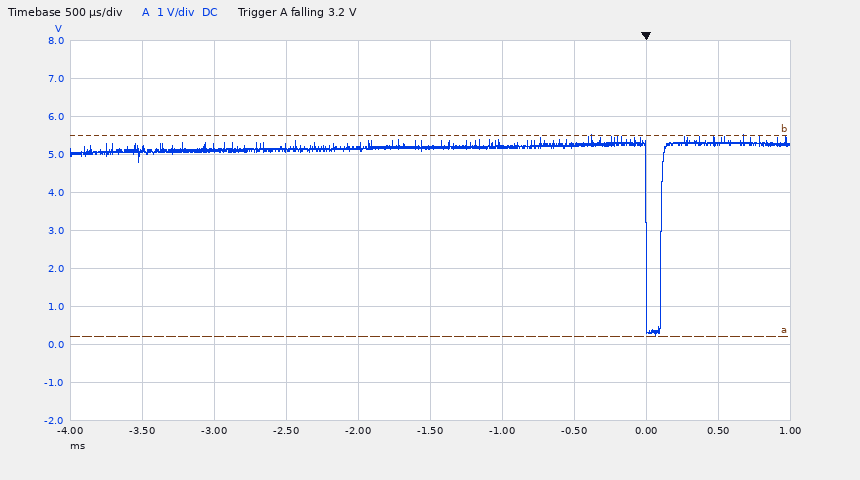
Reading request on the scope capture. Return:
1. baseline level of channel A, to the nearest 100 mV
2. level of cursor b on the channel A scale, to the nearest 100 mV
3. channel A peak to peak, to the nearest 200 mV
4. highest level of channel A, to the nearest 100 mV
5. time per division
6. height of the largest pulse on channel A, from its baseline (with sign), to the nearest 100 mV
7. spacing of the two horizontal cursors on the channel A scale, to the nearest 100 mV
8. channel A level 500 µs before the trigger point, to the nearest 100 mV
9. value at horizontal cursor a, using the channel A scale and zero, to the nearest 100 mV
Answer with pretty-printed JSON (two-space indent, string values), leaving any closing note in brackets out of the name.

{
  "baseline level of channel A, to the nearest 100 mV": "5.2 V",
  "level of cursor b on the channel A scale, to the nearest 100 mV": "5.5 V",
  "channel A peak to peak, to the nearest 200 mV": "5.2 V",
  "highest level of channel A, to the nearest 100 mV": "5.5 V",
  "time per division": "500 µs",
  "height of the largest pulse on channel A, from its baseline (with sign), to the nearest 100 mV": "-4.9 V",
  "spacing of the two horizontal cursors on the channel A scale, to the nearest 100 mV": "5.3 V",
  "channel A level 500 µs before the trigger point, to the nearest 100 mV": "5.2 V",
  "value at horizontal cursor a, using the channel A scale and zero, to the nearest 100 mV": "200 mV"
}
